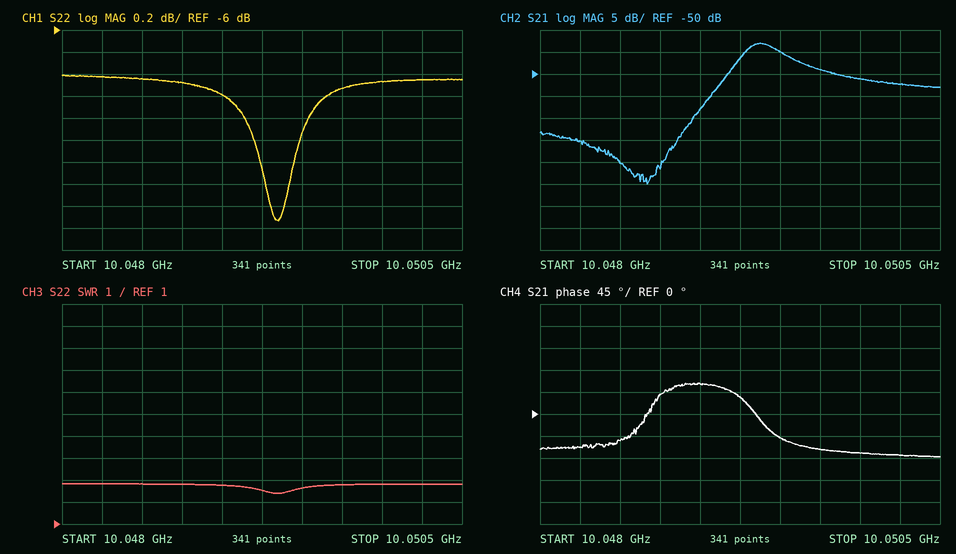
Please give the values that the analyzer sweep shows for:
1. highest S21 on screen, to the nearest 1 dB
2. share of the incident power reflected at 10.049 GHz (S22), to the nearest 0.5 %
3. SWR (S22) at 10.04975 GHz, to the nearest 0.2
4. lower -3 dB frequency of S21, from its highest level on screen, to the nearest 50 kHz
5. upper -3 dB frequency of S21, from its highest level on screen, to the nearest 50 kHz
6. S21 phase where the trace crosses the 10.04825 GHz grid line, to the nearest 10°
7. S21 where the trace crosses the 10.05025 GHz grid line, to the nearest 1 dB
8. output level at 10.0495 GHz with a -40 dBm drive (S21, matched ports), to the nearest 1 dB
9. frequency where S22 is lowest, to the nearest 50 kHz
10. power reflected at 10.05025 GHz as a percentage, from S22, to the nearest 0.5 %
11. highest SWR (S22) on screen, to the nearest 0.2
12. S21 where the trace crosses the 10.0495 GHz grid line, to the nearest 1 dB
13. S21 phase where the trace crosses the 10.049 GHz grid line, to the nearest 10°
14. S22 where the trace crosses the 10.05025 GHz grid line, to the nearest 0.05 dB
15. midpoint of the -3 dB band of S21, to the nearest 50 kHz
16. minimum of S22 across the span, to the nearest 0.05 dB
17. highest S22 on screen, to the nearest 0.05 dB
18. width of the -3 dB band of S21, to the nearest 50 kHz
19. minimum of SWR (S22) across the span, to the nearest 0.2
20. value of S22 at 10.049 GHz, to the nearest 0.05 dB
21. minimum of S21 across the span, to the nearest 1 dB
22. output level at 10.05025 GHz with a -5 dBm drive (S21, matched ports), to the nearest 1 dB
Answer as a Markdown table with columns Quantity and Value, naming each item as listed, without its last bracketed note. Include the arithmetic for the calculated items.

| Quantity | Value |
|---|---|
| highest S21 on screen, to the nearest 1 dB | -43 dB |
| share of the incident power reflected at 10.049 GHz (S22), to the nearest 0.5 % | 10^(-6.6/10) ≈ 21.9 %, so 22.0 % to the nearest 0.5 % |
| SWR (S22) at 10.04975 GHz, to the nearest 0.2 | 2.8 |
| lower -3 dB frequency of S21, from its highest level on screen, to the nearest 50 kHz | 10.04925 GHz |
| upper -3 dB frequency of S21, from its highest level on screen, to the nearest 50 kHz | 10.04955 GHz |
| S21 phase where the trace crosses the 10.04825 GHz grid line, to the nearest 10° | -70° |
| S21 where the trace crosses the 10.05025 GHz grid line, to the nearest 1 dB | -52 dB |
| output level at 10.0495 GHz with a -40 dBm drive (S21, matched ports), to the nearest 1 dB | -40 dBm + (-45 dB) = -85 dBm |
| frequency where S22 is lowest, to the nearest 50 kHz | 10.04935 GHz |
| power reflected at 10.05025 GHz as a percentage, from S22, to the nearest 0.5 % | 10^(-6.45/10) ≈ 22.6 %, so 22.5 % to the nearest 0.5 % |
| highest SWR (S22) on screen, to the nearest 0.2 | 2.8 |
| S21 where the trace crosses the 10.0495 GHz grid line, to the nearest 1 dB | -45 dB |
| S21 phase where the trace crosses the 10.049 GHz grid line, to the nearest 10° | 60° |
| S22 where the trace crosses the 10.05025 GHz grid line, to the nearest 0.05 dB | -6.45 dB |
| midpoint of the -3 dB band of S21, to the nearest 50 kHz | 10.04940 GHz |
| minimum of S22 across the span, to the nearest 0.05 dB | -7.75 dB |
| highest S22 on screen, to the nearest 0.05 dB | -6.40 dB |
| width of the -3 dB band of S21, to the nearest 50 kHz | 10.04955 GHz − 10.04925 GHz = 300 kHz |
| minimum of SWR (S22) across the span, to the nearest 0.2 | 2.4 |
| value of S22 at 10.049 GHz, to the nearest 0.05 dB | -6.60 dB |
| minimum of S21 across the span, to the nearest 1 dB | -75 dB |
| output level at 10.05025 GHz with a -5 dBm drive (S21, matched ports), to the nearest 1 dB | -5 dBm + (-52 dB) = -57 dBm |
